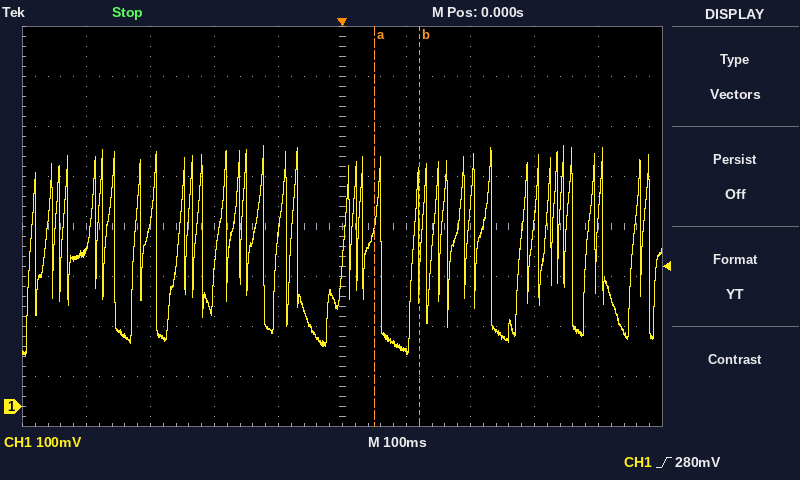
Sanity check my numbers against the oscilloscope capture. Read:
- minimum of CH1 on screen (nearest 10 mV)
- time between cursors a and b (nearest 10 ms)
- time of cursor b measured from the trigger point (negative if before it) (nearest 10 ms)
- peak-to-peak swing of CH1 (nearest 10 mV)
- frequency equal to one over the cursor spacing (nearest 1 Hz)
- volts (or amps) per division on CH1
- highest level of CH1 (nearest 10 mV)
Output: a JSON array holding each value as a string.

["100 mV", "70 ms", "+120 ms", "420 mV", "14 Hz", "100 mV", "520 mV"]
